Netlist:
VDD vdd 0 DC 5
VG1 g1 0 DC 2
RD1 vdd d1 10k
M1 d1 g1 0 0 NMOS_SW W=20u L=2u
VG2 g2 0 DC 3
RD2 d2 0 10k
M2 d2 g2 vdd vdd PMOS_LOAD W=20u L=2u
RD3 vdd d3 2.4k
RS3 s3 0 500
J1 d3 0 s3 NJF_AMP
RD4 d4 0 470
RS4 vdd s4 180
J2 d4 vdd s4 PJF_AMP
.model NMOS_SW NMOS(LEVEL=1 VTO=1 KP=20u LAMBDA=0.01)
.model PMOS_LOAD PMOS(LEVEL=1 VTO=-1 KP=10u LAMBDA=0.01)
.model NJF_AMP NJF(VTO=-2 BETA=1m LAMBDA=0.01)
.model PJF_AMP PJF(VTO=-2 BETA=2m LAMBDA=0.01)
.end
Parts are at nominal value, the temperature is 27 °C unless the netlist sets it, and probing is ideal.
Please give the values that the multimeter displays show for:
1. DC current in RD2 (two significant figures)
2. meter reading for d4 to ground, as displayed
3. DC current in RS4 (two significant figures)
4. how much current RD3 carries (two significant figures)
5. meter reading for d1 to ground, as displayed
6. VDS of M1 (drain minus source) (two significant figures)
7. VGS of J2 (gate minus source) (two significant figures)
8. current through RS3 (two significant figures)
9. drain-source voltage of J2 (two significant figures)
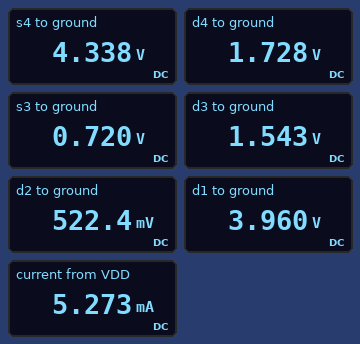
52 µA
1.728 V
3.7 mA
1.4 mA
3.960 V
4.0 V
660 mV
1.4 mA
-2.6 V
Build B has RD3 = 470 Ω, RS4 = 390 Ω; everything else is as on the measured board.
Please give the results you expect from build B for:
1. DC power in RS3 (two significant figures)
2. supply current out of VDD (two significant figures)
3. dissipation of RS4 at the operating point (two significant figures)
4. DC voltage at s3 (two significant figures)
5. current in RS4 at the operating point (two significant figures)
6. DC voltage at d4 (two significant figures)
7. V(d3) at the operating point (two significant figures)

1.2 mW
4.1 mA
2.2 mW
780 mV
2.4 mA
1.1 V
4.3 V
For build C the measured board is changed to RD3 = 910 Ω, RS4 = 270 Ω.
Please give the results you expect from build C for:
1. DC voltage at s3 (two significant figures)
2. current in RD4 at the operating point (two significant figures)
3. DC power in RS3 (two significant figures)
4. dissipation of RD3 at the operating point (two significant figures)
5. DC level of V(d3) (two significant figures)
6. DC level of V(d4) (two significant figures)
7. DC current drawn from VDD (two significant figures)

770 mV
3.0 mA
1.2 mW
2.2 mW
3.6 V
1.4 V
4.7 mA
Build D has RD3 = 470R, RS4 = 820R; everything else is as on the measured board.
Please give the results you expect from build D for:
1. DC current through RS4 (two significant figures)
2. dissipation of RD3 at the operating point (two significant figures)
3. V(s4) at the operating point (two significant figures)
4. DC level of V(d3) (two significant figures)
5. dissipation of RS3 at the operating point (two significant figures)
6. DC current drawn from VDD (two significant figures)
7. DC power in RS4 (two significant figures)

1.4 mA
1.1 mW
3.8 V
4.3 V
1.2 mW
3.1 mA
1.7 mW
